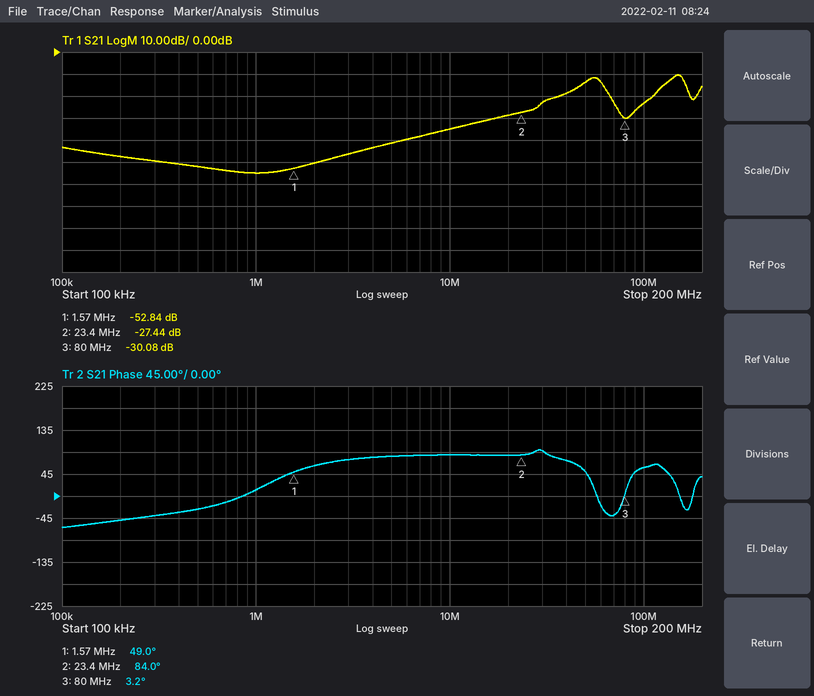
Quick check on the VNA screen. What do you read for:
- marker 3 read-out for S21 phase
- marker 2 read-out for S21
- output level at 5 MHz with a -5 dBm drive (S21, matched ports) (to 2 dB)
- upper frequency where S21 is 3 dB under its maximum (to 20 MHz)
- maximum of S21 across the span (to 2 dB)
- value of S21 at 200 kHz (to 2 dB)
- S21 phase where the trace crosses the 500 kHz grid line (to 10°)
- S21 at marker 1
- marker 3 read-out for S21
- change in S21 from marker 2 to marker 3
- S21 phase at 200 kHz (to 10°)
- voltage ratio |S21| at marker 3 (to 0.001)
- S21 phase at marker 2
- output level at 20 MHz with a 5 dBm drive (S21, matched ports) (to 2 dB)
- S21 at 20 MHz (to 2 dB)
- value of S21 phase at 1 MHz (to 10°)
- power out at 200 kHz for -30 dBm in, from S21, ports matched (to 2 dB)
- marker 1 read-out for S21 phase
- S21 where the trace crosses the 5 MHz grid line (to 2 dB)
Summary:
3.2°
-27.44 dB
-46 dBm
160 MHz
-10 dB
-48 dB
-30°
-52.84 dB
-30.08 dB
-2.64 dB
-50°
0.031
84.0°
-24 dBm
-28 dB
10°
-78 dBm
49.0°
-42 dB
